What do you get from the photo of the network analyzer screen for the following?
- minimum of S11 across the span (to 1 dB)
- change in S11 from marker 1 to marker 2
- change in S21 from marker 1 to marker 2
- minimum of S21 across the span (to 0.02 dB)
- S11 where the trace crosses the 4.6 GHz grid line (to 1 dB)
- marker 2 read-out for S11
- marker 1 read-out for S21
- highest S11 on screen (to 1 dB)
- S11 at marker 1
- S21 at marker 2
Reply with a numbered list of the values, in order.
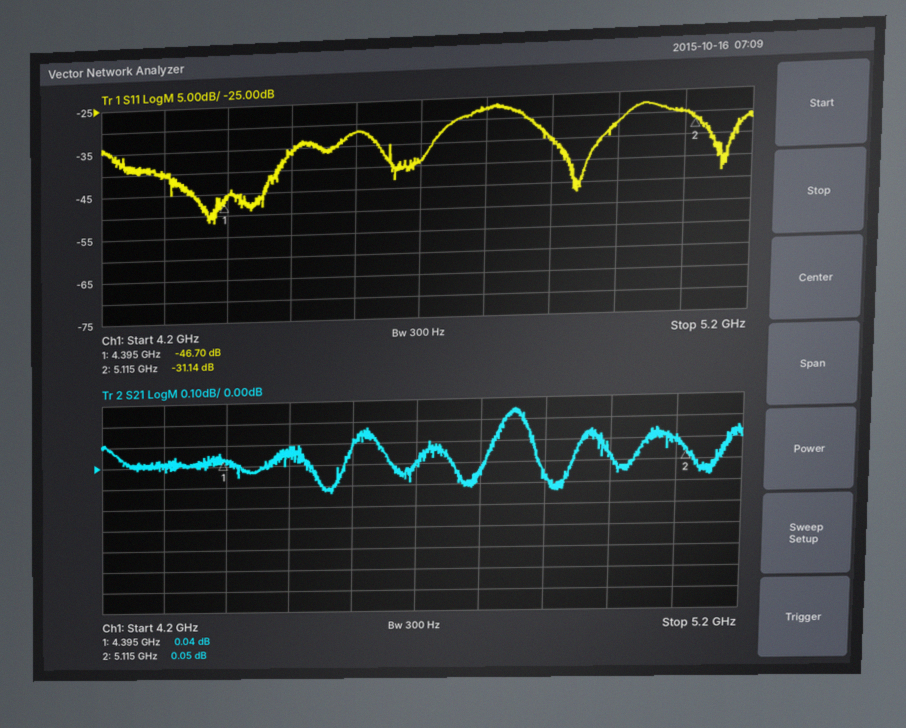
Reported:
1. -52 dB
2. 15.56 dB
3. 0.01 dB
4. -0.14 dB
5. -32 dB
6. -31.14 dB
7. 0.04 dB
8. -27 dB
9. -46.70 dB
10. 0.05 dB
